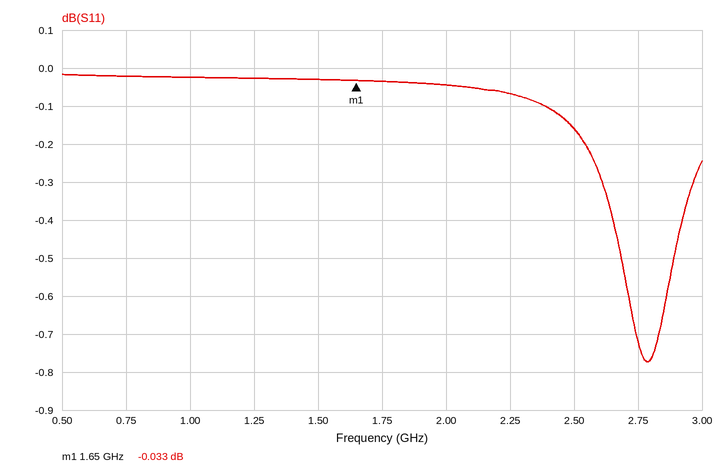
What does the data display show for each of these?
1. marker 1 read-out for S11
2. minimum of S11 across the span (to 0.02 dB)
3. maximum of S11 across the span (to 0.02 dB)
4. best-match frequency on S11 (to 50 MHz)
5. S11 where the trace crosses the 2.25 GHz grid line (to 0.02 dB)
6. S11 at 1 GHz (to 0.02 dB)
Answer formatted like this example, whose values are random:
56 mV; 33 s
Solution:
-0.033 dB; -0.78 dB; -0.02 dB; 2.80 GHz; -0.06 dB; -0.02 dB
